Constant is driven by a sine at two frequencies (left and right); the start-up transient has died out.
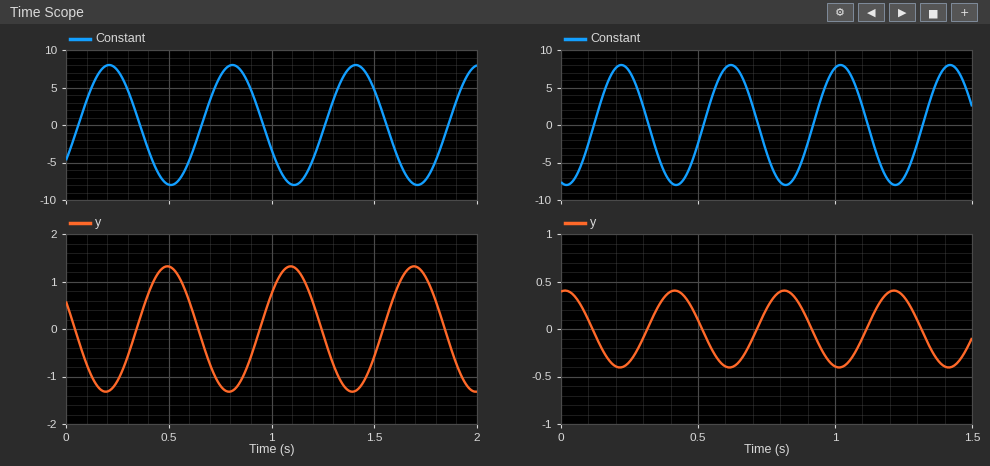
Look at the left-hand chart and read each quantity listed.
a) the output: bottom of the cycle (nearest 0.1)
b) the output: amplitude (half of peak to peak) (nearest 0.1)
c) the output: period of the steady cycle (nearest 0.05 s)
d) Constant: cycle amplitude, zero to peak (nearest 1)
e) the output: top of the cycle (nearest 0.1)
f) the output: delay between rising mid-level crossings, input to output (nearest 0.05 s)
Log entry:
-1.3
1.3
0.60 s
8
1.3
0.30 s
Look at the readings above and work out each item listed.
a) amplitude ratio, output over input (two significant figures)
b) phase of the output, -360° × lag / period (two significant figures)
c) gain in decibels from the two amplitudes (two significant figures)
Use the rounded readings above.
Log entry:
0.16
-180°
-16 dB
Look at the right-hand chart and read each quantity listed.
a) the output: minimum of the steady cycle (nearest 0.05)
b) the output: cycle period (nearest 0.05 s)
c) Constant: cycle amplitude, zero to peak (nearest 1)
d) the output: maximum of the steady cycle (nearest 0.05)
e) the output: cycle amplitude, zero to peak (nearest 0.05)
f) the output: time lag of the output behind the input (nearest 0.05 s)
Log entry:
-0.40
0.40 s
8
0.40
0.40
0.20 s
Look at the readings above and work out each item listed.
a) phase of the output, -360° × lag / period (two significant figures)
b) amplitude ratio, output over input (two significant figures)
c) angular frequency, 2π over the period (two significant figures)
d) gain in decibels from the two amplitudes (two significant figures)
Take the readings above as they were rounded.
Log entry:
-180°
0.050
16 rad/s
-26 dB
